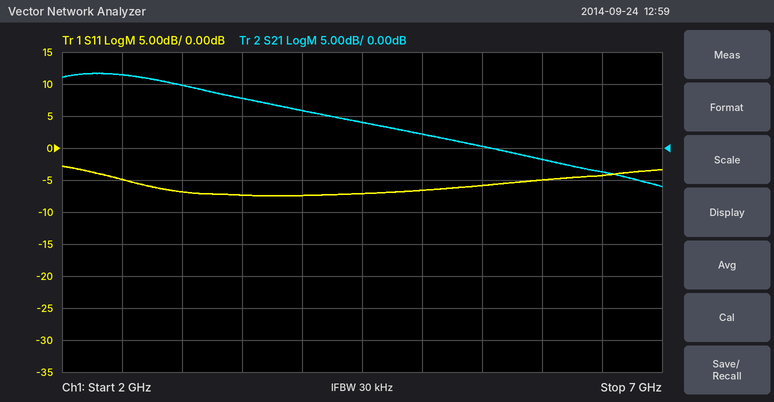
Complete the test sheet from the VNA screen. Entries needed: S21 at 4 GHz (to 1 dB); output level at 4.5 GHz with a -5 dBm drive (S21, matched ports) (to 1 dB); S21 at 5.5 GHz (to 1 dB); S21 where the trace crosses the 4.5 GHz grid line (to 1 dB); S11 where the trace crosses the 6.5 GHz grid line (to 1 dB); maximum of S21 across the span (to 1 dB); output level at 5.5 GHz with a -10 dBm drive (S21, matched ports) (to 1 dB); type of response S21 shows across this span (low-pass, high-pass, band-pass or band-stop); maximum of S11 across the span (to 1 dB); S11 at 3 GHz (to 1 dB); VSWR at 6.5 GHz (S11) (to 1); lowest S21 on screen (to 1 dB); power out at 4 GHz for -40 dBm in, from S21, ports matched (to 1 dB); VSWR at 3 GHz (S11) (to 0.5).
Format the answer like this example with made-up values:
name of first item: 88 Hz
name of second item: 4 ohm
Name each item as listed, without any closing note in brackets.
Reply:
S21 at 4 GHz: 6 dB
output level at 4.5 GHz with a -5 dBm drive (S21, matched ports): -1 dBm
S21 at 5.5 GHz: 0 dB
S21 where the trace crosses the 4.5 GHz grid line: 4 dB
S11 where the trace crosses the 6.5 GHz grid line: -4 dB
maximum of S21 across the span: 12 dB
output level at 5.5 GHz with a -10 dBm drive (S21, matched ports): -10 dBm
type of response S21 shows across this span: low-pass
maximum of S11 across the span: -3 dB
S11 at 3 GHz: -7 dB
VSWR at 6.5 GHz (S11): 4
lowest S21 on screen: -6 dB
power out at 4 GHz for -40 dBm in, from S21, ports matched: -34 dBm
VSWR at 3 GHz (S11): 2.5
